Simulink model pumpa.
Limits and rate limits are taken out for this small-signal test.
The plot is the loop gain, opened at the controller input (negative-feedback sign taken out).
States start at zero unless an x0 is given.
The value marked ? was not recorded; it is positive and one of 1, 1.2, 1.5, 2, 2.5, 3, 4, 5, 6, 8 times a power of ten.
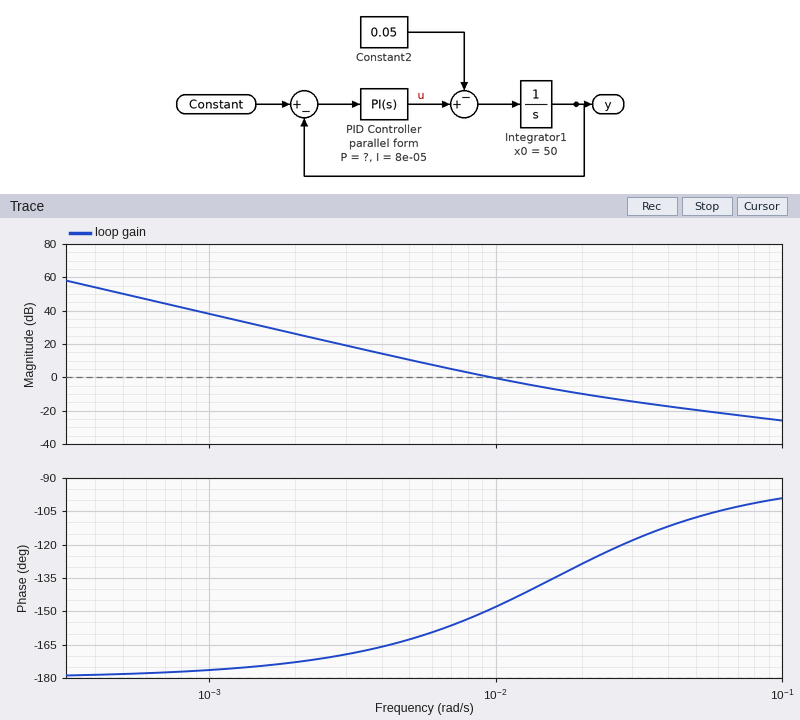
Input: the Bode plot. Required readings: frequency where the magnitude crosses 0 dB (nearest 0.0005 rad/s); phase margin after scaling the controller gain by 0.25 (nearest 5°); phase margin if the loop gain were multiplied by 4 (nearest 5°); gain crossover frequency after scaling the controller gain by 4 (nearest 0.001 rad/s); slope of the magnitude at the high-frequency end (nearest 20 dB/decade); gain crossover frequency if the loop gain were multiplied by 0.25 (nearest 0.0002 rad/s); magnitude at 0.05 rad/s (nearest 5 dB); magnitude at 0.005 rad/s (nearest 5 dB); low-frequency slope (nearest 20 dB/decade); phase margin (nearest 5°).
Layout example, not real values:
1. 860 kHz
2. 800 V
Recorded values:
1. 0.0095 rad/s
2. 15°
3. 55°
4. 0.024 rad/s
5. -20 dB/decade
6. 0.0046 rad/s
7. -20 dB
8. 10 dB
9. -40 dB/decade
10. 30°
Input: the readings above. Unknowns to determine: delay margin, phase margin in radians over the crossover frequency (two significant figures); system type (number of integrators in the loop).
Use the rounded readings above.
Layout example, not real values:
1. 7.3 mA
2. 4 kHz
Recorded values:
1. 55 s
2. 2
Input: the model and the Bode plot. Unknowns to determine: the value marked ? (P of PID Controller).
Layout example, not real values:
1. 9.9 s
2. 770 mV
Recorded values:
1. 0.005
